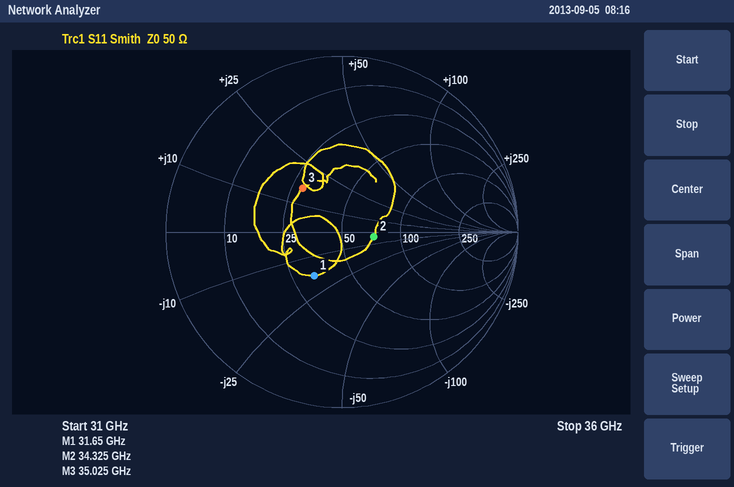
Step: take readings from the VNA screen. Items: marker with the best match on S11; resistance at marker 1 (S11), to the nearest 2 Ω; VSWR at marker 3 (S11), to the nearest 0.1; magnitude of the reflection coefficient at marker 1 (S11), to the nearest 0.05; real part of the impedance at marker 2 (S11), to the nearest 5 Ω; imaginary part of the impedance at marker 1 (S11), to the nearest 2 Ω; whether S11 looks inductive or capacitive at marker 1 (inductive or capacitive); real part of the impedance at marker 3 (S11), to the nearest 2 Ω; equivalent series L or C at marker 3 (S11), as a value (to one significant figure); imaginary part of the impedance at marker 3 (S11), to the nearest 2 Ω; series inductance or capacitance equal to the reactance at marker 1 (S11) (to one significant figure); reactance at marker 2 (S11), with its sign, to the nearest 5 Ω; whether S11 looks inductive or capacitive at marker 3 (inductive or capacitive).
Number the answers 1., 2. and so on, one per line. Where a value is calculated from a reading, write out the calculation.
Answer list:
1. marker 2
2. 32 Ω
3. 2.0
4. 0.30
5. 70 Ω
6. -18 Ω
7. capacitive
8. 28 Ω
9. L = 16 Ω/(2π × 35.025 GHz) ≈ 72.7 pH, so 70 pH to one significant figure
10. +16 Ω
11. C = 1/(2π × 31.65 GHz × 18 Ω) ≈ 279 fF, so 300 fF to one significant figure
12. -5 Ω
13. inductive
